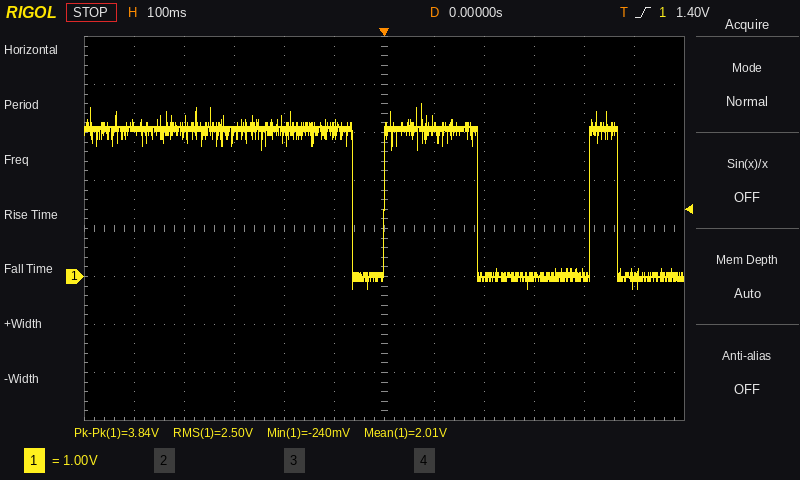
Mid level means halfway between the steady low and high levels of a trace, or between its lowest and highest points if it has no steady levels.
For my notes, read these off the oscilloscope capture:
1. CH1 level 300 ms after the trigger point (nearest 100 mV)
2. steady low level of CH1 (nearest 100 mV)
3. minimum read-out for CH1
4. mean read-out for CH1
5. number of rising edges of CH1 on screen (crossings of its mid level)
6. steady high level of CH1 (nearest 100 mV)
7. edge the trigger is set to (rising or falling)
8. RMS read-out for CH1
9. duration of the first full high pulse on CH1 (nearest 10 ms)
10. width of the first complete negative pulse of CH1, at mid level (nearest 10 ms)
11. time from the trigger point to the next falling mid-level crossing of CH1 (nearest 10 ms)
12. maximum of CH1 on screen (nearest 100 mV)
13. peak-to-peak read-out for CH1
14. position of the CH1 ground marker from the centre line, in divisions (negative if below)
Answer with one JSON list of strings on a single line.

["0.0 V", "0.0 V", "-240 mV", "2.01 V", "2", "3.1 V", "rising", "2.50 V", "190 ms", "60 ms", "190 ms", "3.6 V", "3.84 V", "-1.0 div"]
